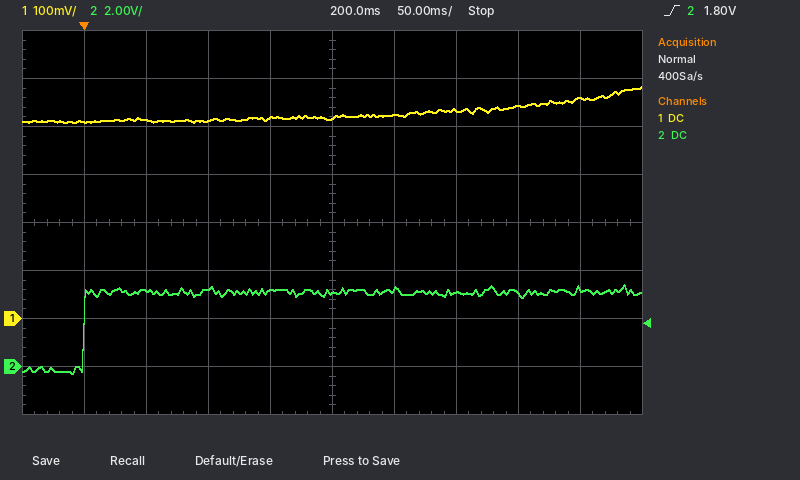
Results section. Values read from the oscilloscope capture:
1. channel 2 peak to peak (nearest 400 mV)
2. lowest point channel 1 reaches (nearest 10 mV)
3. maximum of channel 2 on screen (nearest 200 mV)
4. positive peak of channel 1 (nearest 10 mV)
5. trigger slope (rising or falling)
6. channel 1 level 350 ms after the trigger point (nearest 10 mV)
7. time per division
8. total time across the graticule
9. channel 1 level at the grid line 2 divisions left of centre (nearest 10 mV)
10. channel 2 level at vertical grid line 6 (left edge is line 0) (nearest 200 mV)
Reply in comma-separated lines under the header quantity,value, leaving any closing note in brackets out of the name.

quantity,value
channel 2 peak to peak,3.6 V
lowest point channel 1 reaches,410 mV
maximum of channel 2 on screen,3.4 V
positive peak of channel 1,480 mV
trigger slope,rising
channel 1 level 350 ms after the trigger point,440 mV
time per division,50 ms
total time across the graticule,500 ms
channel 1 level at the grid line 2 divisions left of centre,410 mV
channel 2 level at vertical grid line 6 (left edge is line 0),3.2 V
